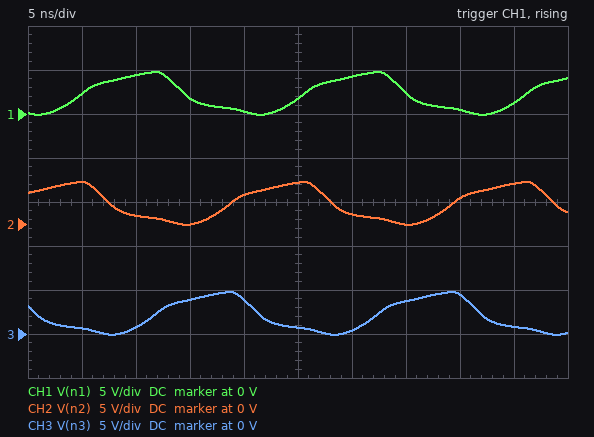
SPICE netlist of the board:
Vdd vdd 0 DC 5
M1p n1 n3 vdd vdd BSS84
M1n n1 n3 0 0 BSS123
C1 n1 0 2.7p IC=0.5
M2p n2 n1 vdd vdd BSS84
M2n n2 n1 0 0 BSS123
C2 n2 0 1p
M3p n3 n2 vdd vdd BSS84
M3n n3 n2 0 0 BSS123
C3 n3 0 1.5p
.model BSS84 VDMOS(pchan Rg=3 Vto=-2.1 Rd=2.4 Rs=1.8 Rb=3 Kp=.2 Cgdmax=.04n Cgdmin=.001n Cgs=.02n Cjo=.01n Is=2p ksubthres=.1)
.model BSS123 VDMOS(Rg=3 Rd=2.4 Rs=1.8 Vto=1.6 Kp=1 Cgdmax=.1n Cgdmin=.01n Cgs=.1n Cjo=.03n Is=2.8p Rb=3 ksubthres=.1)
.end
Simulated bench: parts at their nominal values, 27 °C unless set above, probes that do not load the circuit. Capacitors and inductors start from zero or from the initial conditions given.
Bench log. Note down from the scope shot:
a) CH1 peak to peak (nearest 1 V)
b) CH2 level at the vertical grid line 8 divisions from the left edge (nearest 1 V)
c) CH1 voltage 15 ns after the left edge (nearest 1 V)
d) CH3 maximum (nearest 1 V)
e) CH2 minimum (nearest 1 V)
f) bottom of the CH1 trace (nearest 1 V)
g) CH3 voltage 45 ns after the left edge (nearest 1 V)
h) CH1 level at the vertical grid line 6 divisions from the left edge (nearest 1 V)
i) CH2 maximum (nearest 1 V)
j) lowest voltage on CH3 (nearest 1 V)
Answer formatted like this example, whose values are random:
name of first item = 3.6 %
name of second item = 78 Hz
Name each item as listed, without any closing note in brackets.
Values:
CH1 peak to peak = 5 V
CH2 level at the vertical grid line 8 divisions from the left edge = 3 V
CH1 voltage 15 ns after the left edge = 2 V
CH3 maximum = 5 V
CH2 minimum = 0 V
bottom of the CH1 trace = 0 V
CH3 voltage 45 ns after the left edge = 1 V
CH1 level at the vertical grid line 6 divisions from the left edge = 4 V
CH2 maximum = 5 V
lowest voltage on CH3 = 0 V
